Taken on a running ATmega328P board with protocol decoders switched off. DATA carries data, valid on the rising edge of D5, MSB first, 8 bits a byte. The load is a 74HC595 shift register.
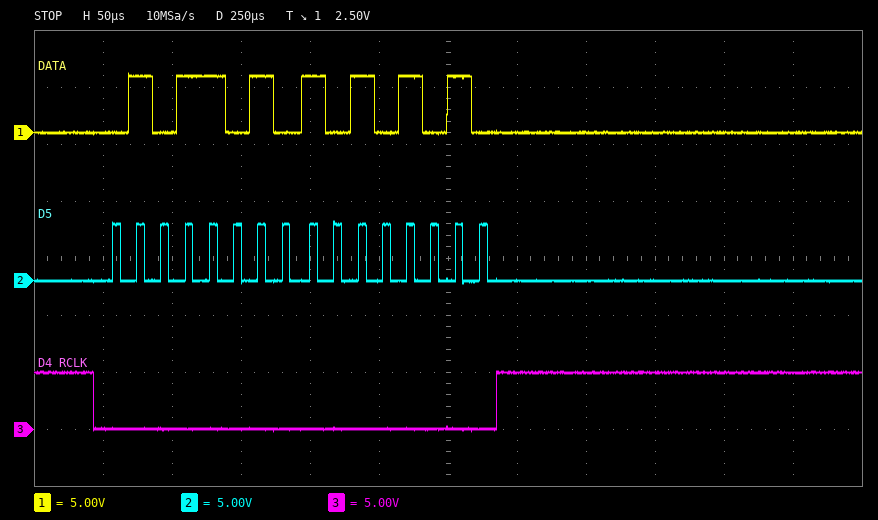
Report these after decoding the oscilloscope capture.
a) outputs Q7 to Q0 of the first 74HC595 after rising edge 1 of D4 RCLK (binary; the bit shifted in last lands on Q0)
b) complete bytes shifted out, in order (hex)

10101010
5A AA
